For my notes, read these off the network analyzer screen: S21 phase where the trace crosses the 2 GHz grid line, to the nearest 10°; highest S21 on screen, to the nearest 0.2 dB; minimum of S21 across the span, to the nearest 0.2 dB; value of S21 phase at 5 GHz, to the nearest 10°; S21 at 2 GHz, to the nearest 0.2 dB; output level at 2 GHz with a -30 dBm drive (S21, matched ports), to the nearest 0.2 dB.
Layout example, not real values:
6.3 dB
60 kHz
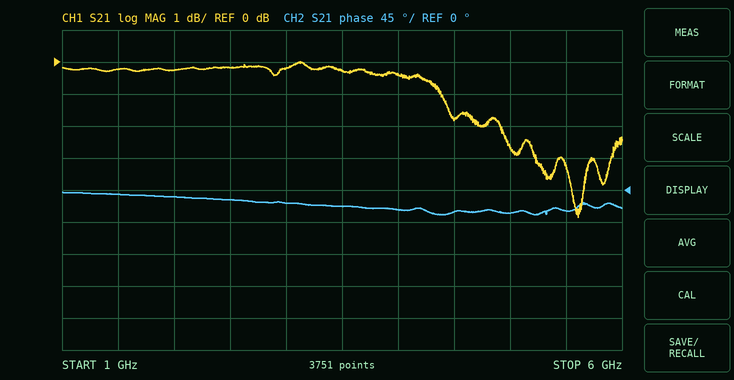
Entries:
-10°
0.0 dB
-4.8 dB
-30°
-0.2 dB
-30.2 dBm
